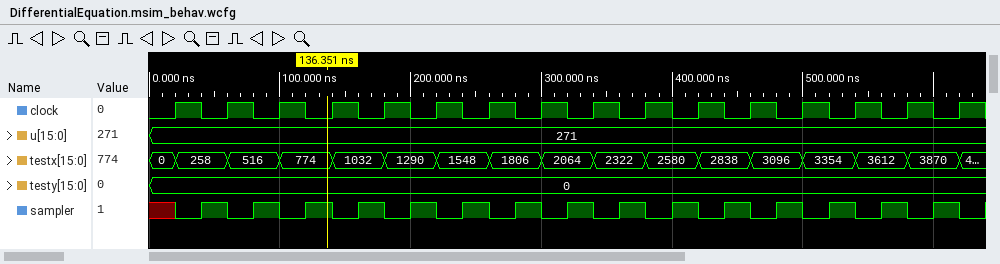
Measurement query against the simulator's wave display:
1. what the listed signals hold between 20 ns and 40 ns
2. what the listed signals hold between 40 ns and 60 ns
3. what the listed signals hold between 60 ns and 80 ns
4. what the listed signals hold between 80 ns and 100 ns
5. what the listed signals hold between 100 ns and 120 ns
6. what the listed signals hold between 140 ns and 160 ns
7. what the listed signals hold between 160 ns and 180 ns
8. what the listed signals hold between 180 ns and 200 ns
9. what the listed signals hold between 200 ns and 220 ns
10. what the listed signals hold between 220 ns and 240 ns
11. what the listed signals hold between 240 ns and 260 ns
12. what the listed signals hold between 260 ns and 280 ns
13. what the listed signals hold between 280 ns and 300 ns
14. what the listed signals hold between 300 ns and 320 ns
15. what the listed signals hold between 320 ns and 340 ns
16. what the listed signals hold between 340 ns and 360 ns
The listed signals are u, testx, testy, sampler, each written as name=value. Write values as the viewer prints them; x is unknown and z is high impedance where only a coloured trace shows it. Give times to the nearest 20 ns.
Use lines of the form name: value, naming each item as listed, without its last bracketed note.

what the listed signals hold between 20 ns and 40 ns: u=271, testx=258, testy=0, sampler=0
what the listed signals hold between 40 ns and 60 ns: u=271, testx=258, testy=0, sampler=1
what the listed signals hold between 60 ns and 80 ns: u=271, testx=516, testy=0, sampler=0
what the listed signals hold between 80 ns and 100 ns: u=271, testx=516, testy=0, sampler=1
what the listed signals hold between 100 ns and 120 ns: u=271, testx=774, testy=0, sampler=0
what the listed signals hold between 140 ns and 160 ns: u=271, testx=1032, testy=0, sampler=0
what the listed signals hold between 160 ns and 180 ns: u=271, testx=1032, testy=0, sampler=1
what the listed signals hold between 180 ns and 200 ns: u=271, testx=1290, testy=0, sampler=0
what the listed signals hold between 200 ns and 220 ns: u=271, testx=1290, testy=0, sampler=1
what the listed signals hold between 220 ns and 240 ns: u=271, testx=1548, testy=0, sampler=0
what the listed signals hold between 240 ns and 260 ns: u=271, testx=1548, testy=0, sampler=1
what the listed signals hold between 260 ns and 280 ns: u=271, testx=1806, testy=0, sampler=0
what the listed signals hold between 280 ns and 300 ns: u=271, testx=1806, testy=0, sampler=1
what the listed signals hold between 300 ns and 320 ns: u=271, testx=2064, testy=0, sampler=0
what the listed signals hold between 320 ns and 340 ns: u=271, testx=2064, testy=0, sampler=1
what the listed signals hold between 340 ns and 360 ns: u=271, testx=2322, testy=0, sampler=0
